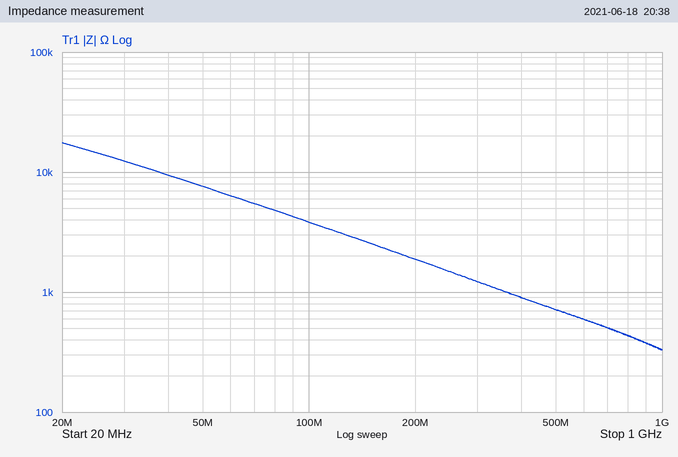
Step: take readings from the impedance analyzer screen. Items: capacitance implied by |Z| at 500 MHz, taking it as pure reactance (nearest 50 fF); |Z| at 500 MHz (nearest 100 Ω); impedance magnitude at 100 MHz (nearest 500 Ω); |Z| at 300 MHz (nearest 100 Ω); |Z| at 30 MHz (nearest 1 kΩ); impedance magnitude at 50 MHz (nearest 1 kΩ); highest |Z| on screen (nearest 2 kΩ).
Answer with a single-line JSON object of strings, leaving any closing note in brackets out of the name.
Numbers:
{"capacitance implied by |Z| at 500 MHz, taking it as pure reactance": "450 fF", "|Z| at 500 MHz": "700 Ω", "impedance magnitude at 100 MHz": "4.0 kΩ", "|Z| at 300 MHz": "1.2 kΩ", "|Z| at 30 MHz": "12 kΩ", "impedance magnitude at 50 MHz": "8 kΩ", "highest |Z| on screen": "18 kΩ"}
